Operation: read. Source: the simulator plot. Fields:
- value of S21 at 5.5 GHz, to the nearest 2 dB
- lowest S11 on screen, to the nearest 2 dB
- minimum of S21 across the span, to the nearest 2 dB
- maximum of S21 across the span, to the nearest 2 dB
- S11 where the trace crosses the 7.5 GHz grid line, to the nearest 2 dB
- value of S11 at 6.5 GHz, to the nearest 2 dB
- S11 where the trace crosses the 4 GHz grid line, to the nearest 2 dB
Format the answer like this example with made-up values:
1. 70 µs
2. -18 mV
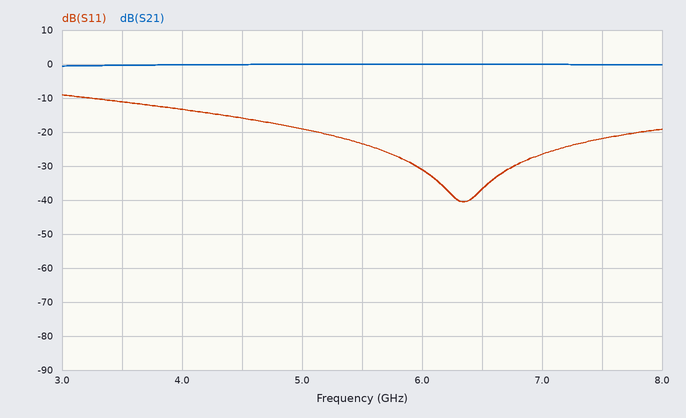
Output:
1. 0 dB
2. -40 dB
3. 0 dB
4. 0 dB
5. -22 dB
6. -36 dB
7. -14 dB
